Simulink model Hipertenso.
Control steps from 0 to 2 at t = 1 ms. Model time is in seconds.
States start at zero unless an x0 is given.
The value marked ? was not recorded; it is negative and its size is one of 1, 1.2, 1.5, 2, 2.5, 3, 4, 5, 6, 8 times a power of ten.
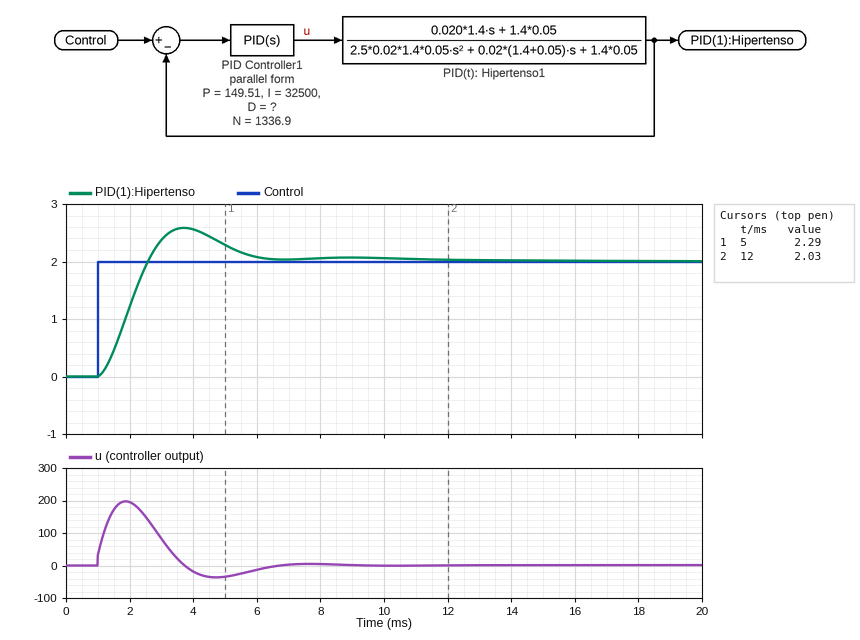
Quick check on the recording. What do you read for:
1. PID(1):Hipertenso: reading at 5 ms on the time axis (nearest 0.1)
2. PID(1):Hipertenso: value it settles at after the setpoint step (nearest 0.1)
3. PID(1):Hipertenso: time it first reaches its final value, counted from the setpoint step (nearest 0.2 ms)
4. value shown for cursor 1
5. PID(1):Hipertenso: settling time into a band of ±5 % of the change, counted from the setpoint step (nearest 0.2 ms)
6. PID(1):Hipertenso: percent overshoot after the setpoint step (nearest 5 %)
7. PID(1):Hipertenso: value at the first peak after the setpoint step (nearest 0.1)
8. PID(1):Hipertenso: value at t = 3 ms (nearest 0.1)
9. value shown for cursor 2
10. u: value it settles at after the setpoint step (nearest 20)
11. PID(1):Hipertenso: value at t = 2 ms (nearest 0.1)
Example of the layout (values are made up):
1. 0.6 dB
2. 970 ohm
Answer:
1. 2.3
2. 2.0
3. 1.6 ms
4. 2.29
5. 4.8 ms
6. 30 %
7. 2.6
8. 2.4
9. 2.03
10. 0
11. 1.2
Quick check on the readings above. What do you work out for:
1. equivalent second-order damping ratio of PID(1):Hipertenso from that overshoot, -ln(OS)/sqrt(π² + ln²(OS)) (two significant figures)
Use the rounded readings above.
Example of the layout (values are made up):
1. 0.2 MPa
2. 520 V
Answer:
1. 0.36
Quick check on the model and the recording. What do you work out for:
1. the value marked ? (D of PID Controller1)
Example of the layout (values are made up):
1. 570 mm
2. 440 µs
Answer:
1. -0.1
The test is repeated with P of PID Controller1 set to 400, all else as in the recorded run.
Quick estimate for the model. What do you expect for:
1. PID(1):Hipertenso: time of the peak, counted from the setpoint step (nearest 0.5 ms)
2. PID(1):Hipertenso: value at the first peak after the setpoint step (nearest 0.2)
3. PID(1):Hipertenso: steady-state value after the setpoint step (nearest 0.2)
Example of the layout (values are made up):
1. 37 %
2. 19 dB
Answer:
1. 1.5 ms
2. 2.2
3. 2.0
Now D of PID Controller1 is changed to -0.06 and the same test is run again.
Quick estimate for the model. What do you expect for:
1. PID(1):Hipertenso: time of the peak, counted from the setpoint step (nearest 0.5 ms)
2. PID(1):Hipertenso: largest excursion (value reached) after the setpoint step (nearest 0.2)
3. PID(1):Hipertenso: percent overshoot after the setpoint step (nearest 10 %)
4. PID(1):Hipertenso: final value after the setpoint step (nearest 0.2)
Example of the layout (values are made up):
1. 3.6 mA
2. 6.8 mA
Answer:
1. 3.0 ms
2. 2.4
3. 20 %
4. 2.0
